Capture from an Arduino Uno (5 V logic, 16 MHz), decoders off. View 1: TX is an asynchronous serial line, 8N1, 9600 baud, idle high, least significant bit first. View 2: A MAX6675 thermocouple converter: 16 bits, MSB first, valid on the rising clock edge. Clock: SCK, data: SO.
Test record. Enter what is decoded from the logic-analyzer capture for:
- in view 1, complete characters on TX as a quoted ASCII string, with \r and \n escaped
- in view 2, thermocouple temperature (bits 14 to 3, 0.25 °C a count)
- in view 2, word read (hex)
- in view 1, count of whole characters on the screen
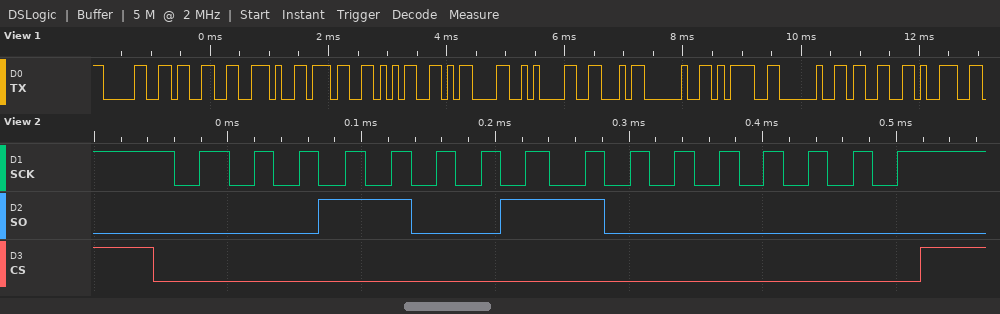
"03.75\r\nF = 39"
204.00 °C
0x1980
13
